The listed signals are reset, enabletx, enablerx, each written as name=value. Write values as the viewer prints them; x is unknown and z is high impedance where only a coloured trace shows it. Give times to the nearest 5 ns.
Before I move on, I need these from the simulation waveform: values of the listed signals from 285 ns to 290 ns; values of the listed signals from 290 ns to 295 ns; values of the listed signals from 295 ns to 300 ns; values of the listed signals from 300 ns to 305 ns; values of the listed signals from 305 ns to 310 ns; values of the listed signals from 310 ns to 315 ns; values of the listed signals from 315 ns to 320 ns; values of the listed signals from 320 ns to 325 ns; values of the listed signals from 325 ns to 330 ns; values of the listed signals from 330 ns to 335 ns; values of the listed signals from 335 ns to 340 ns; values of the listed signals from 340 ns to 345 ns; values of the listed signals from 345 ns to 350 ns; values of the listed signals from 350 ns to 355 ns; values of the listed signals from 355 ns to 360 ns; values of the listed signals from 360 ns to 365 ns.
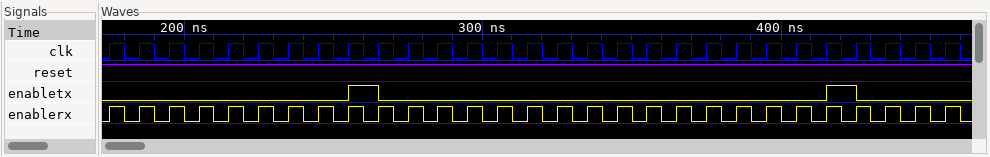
reset=1, enabletx=0, enablerx=1
reset=1, enabletx=0, enablerx=0
reset=1, enabletx=0, enablerx=1
reset=1, enabletx=0, enablerx=0
reset=1, enabletx=0, enablerx=1
reset=1, enabletx=0, enablerx=0
reset=1, enabletx=0, enablerx=1
reset=1, enabletx=0, enablerx=0
reset=1, enabletx=0, enablerx=1
reset=1, enabletx=0, enablerx=0
reset=1, enabletx=0, enablerx=1
reset=1, enabletx=0, enablerx=0
reset=1, enabletx=0, enablerx=1
reset=1, enabletx=0, enablerx=0
reset=1, enabletx=0, enablerx=1
reset=1, enabletx=0, enablerx=0
